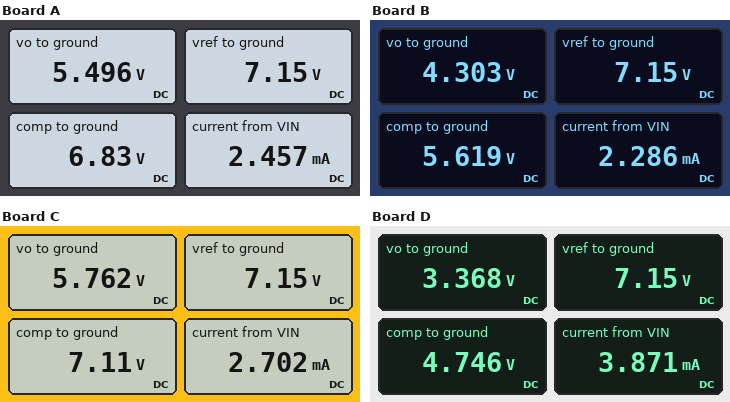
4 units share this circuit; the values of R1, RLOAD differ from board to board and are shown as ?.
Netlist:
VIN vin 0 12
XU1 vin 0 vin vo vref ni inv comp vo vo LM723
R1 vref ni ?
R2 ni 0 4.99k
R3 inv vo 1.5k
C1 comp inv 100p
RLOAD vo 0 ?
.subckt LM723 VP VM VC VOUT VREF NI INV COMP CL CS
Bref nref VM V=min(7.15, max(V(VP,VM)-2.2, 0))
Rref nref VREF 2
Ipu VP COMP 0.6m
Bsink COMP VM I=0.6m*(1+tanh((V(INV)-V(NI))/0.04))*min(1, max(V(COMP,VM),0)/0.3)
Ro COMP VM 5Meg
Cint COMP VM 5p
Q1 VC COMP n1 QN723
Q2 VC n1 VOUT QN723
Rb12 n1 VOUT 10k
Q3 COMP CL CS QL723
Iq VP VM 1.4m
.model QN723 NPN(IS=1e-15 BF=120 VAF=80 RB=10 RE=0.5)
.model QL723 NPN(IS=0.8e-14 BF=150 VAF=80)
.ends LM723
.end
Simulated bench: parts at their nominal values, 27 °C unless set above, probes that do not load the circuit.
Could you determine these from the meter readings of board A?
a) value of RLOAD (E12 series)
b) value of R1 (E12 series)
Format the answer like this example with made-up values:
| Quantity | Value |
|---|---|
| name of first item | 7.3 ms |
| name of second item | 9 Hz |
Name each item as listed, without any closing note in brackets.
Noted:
| Quantity | Value |
|---|---|
| value of RLOAD | 12 kΩ |
| value of R1 | 1.5 kΩ |
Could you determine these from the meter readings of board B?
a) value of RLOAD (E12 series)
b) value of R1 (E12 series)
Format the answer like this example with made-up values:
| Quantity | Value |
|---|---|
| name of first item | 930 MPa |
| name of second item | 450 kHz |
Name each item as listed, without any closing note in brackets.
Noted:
| Quantity | Value |
|---|---|
| value of RLOAD | 15 kΩ |
| value of R1 | 3.3 kΩ |
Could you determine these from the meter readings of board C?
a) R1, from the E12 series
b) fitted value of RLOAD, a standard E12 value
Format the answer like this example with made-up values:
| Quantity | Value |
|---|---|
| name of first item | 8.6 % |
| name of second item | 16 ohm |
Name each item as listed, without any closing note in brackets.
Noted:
| Quantity | Value |
|---|---|
| R1, from the E12 series | 1.2 kΩ |
| fitted value of RLOAD, a standard E12 value | 8.2 kΩ |
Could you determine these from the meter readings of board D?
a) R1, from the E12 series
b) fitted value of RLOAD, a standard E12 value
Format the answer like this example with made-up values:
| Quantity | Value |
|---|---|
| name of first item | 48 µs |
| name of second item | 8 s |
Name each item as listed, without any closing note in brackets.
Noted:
| Quantity | Value |
|---|---|
| R1, from the E12 series | 5.6 kΩ |
| fitted value of RLOAD, a standard E12 value | 1.8 kΩ |
